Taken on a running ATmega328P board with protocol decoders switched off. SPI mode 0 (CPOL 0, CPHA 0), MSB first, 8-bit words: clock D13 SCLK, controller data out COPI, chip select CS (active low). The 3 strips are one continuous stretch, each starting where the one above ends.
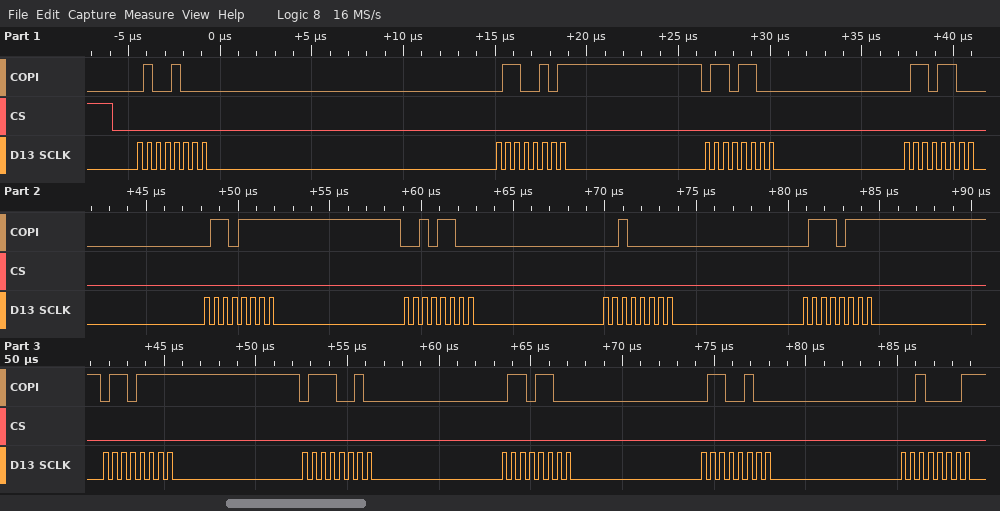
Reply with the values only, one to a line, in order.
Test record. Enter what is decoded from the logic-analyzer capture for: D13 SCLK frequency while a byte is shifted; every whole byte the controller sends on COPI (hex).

2 MHz
48 65 6C 6C 6F 2C 20 77 6F 72 6C 64 21
